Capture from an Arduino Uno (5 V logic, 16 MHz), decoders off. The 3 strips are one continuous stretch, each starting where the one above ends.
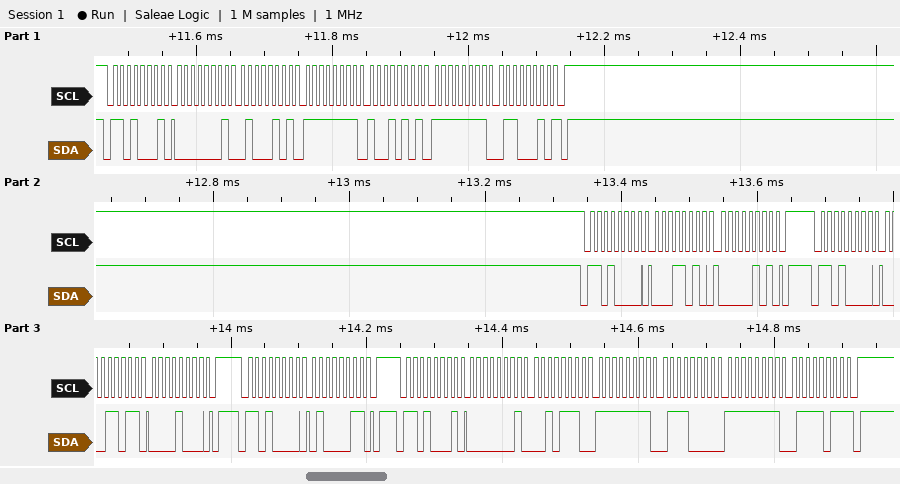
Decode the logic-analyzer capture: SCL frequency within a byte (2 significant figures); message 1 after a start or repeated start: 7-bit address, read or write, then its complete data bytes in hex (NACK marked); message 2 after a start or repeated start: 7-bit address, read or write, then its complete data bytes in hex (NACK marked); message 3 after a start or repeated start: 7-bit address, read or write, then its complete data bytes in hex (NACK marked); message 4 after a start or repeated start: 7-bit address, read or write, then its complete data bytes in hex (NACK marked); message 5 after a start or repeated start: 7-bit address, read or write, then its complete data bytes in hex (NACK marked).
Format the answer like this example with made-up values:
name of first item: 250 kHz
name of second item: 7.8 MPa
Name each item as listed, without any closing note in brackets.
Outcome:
SCL frequency within a byte: 100 kHz
message 1 after a start or repeated start: 7-bit address, read or write, then its complete data bytes in hex: 0x68 read: 01 45 FF 95 FF 62 NACK
message 2 after a start or repeated start: 7-bit address, read or write, then its complete data bytes in hex: 0x68 write: 1A 05
message 3 after a start or repeated start: 7-bit address, read or write, then its complete data bytes in hex: 0x68 write: 1B 08
message 4 after a start or repeated start: 7-bit address, read or write, then its complete data bytes in hex: 0x68 write: 43
message 5 after a start or repeated start: 7-bit address, read or write, then its complete data bytes in hex: 0x68 read: 01 2E FF 70 FF 7B NACK
